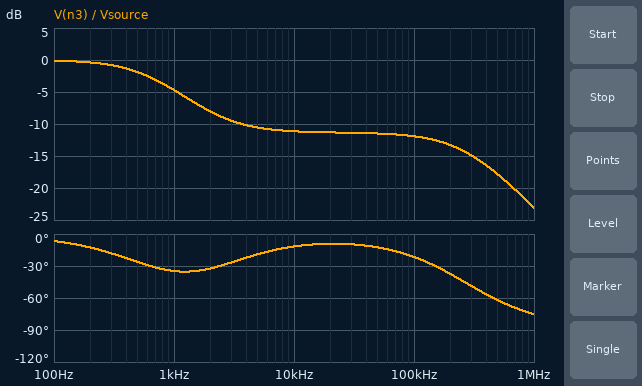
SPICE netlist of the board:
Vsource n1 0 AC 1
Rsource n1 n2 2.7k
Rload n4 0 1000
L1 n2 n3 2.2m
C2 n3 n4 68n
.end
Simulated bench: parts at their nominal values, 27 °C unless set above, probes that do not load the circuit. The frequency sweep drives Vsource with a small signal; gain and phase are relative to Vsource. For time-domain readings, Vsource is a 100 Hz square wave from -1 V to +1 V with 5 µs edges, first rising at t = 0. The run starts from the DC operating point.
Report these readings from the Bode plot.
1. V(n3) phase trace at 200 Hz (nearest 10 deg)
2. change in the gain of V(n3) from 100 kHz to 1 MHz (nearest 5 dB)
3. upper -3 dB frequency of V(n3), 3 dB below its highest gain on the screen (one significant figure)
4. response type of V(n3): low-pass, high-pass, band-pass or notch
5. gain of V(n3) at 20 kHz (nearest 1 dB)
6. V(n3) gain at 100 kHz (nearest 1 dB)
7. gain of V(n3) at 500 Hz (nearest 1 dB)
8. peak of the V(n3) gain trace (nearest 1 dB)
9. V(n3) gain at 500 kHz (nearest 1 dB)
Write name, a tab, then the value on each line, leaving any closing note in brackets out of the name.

V(n3) phase trace at 200 Hz	-10 deg
change in the gain of V(n3) from 100 kHz to 1 MHz	-10 dB
upper -3 dB frequency of V(n3), 3 dB below its highest gain on the screen	700 Hz
response type of V(n3): low-pass, high-pass, band-pass or notch	low-pass
gain of V(n3) at 20 kHz	-11 dB
V(n3) gain at 100 kHz	-12 dB
gain of V(n3) at 500 Hz	-2 dB
peak of the V(n3) gain trace	0 dB
V(n3) gain at 500 kHz	-18 dB
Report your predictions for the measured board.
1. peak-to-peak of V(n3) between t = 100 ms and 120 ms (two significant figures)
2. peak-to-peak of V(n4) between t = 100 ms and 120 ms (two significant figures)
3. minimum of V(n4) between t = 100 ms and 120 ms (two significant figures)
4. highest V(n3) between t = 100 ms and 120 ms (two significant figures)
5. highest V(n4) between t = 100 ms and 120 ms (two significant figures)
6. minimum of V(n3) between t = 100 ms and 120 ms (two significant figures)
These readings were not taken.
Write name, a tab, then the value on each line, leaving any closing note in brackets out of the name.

peak-to-peak of V(n3) between t = 100 ms and 120 ms	2.0 V
peak-to-peak of V(n4) between t = 100 ms and 120 ms	1.1 V
minimum of V(n4) between t = 100 ms and 120 ms	-530 mV
highest V(n3) between t = 100 ms and 120 ms	1.0 V
highest V(n4) between t = 100 ms and 120 ms	530 mV
minimum of V(n3) between t = 100 ms and 120 ms	-1.0 V
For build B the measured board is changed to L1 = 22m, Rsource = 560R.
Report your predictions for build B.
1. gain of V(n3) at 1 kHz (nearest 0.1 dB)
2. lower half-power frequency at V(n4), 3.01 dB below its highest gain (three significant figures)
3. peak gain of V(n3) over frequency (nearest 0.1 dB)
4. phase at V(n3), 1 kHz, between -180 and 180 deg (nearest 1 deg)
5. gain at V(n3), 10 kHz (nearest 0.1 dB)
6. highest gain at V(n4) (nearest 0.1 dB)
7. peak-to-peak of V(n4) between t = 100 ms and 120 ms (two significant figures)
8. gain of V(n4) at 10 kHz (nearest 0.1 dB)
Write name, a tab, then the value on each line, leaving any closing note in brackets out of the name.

gain of V(n3) at 1 kHz	-0.5 dB
lower half-power frequency at V(n4), 3.01 dB below its highest gain	1.34 kHz
peak gain of V(n3) over frequency	0 dB
phase at V(n3), 1 kHz, between -180 and 180 deg	-12 deg
gain at V(n3), 10 kHz	-5.5 dB
highest gain at V(n4)	-3.9 dB
peak-to-peak of V(n4) between t = 100 ms and 120 ms	2.1 V
gain of V(n4) at 10 kHz	-5.7 dB
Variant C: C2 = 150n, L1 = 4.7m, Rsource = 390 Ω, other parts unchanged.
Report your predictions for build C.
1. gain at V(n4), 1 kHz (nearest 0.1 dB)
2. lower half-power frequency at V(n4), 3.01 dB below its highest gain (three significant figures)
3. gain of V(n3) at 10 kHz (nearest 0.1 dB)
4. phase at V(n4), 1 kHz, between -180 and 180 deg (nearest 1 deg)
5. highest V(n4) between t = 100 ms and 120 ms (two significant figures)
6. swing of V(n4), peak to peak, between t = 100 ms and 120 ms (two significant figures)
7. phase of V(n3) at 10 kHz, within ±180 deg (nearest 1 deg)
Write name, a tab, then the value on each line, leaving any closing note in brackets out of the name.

gain at V(n4), 1 kHz	-4.8 dB
lower half-power frequency at V(n4), 3.01 dB below its highest gain	751 Hz
gain of V(n3) at 10 kHz	-2.9 dB
phase at V(n4), 1 kHz, between -180 and 180 deg	37 deg
highest V(n4) between t = 100 ms and 120 ms	1.4 V
swing of V(n4), peak to peak, between t = 100 ms and 120 ms	2.7 V
phase of V(n3) at 10 kHz, within ±180 deg	-14 deg
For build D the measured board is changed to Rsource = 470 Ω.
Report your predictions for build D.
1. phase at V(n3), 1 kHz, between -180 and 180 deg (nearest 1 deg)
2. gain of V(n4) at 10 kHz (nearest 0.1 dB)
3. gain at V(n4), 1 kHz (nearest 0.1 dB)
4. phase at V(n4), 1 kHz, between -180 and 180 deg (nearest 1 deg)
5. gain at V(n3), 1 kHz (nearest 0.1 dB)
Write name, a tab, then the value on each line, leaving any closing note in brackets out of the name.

phase at V(n3), 1 kHz, between -180 and 180 deg	-9 deg
gain of V(n4) at 10 kHz	-3.4 dB
gain at V(n4), 1 kHz	-8.8 dB
phase at V(n4), 1 kHz, between -180 and 180 deg	58 deg
gain at V(n3), 1 kHz	-0.7 dB
